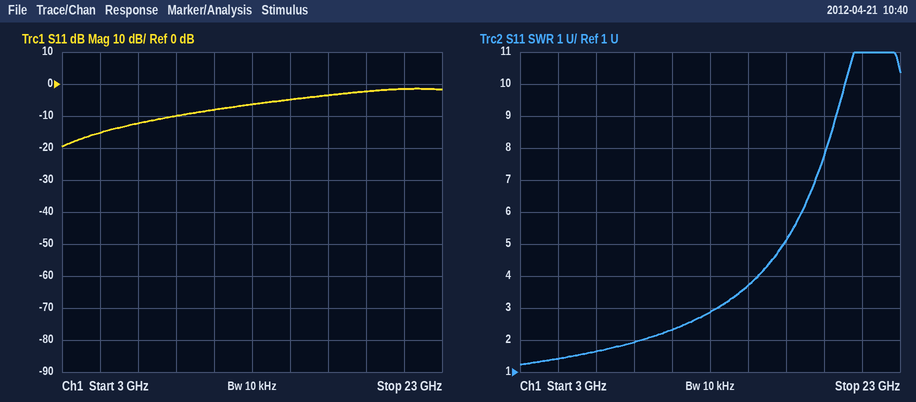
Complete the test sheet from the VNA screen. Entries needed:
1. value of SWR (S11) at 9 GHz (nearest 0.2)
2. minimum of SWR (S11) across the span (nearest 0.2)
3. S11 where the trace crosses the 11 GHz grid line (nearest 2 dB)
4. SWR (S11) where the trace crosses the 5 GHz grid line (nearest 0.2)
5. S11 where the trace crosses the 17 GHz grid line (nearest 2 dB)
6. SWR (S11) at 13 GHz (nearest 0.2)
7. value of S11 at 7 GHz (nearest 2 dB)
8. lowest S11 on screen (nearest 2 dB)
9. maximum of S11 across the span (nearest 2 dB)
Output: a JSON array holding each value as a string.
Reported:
["2.0", "1.2", "-8 dB", "1.4", "-4 dB", "2.8", "-12 dB", "-20 dB", "-2 dB"]
